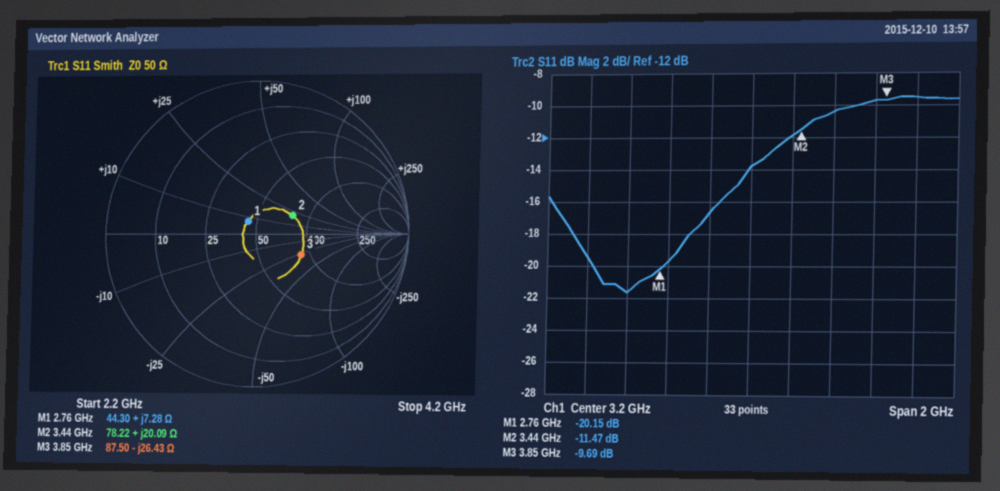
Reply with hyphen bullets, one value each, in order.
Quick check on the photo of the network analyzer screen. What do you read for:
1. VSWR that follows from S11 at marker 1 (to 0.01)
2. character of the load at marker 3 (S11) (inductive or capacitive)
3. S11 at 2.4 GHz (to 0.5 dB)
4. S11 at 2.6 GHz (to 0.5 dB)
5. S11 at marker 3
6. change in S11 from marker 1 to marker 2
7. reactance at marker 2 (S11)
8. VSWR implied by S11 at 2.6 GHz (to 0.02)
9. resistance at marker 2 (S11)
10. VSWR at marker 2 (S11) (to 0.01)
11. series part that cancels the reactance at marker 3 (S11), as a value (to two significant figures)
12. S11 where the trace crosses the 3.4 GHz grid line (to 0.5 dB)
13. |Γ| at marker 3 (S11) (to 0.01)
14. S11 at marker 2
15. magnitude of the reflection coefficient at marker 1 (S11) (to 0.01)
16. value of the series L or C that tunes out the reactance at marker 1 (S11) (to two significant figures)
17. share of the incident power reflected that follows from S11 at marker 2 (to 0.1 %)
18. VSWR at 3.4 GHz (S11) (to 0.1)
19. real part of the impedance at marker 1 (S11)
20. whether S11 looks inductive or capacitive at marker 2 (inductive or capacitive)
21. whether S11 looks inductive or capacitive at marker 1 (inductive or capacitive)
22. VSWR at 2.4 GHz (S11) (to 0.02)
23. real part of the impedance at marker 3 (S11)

- 1.22
- capacitive
- -19.5 dB
- -21.5 dB
- -9.69 dB
- 8.68 dB
- +20.09 Ω
- 1.18
- 78.22 Ω
- 1.73
- 1.1 nH
- -12.0 dB
- 0.33
- -11.47 dB
- 0.10
- 7.9 pF
- 7.1 %
- 1.7
- 44.30 Ω
- inductive
- inductive
- 1.24
- 87.50 Ω
